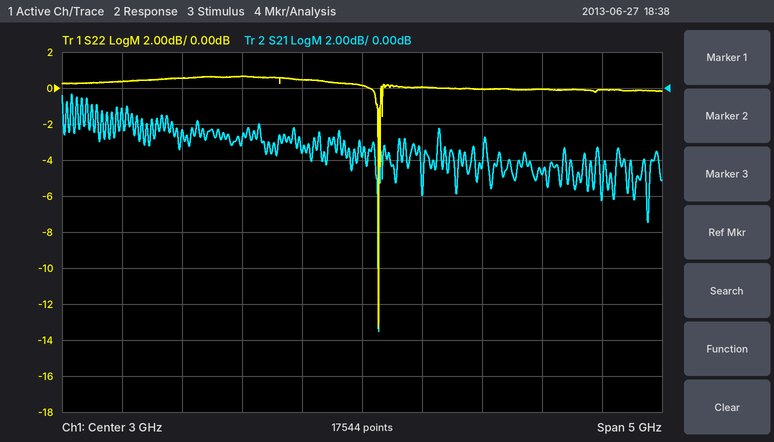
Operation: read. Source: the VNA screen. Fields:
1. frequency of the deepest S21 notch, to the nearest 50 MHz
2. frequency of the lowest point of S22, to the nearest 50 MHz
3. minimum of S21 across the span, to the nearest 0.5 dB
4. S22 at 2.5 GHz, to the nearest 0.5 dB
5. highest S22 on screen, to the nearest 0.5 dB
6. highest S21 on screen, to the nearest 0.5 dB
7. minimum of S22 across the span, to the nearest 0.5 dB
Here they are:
3.15 GHz
3.15 GHz
-13.5 dB
0.5 dB
0.5 dB
-0.5 dB
-13.5 dB
